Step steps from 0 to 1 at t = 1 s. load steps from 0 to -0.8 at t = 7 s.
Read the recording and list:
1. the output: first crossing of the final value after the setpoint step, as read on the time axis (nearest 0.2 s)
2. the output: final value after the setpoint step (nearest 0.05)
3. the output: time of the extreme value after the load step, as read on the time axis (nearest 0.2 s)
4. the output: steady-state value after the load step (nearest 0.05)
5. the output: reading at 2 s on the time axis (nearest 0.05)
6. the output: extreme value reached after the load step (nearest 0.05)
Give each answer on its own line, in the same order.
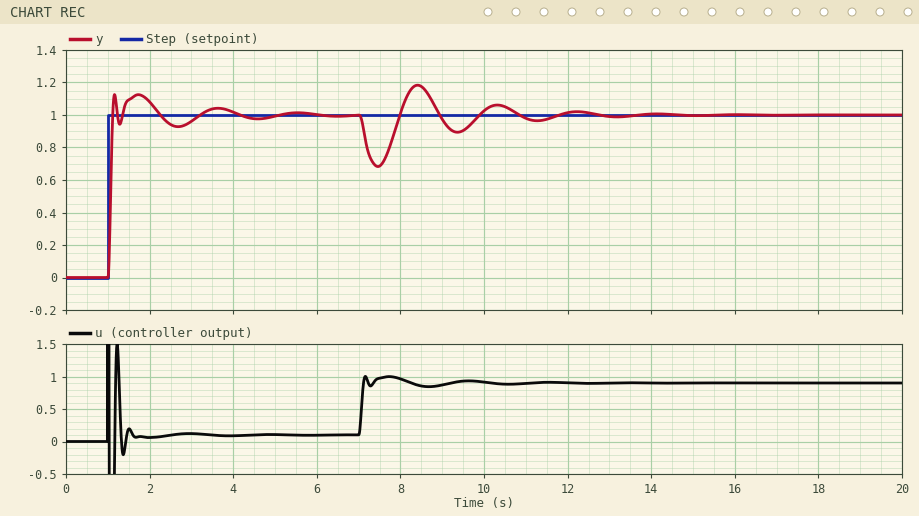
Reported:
1.2 s
1.00
7.4 s
1.00
1.10
0.70
